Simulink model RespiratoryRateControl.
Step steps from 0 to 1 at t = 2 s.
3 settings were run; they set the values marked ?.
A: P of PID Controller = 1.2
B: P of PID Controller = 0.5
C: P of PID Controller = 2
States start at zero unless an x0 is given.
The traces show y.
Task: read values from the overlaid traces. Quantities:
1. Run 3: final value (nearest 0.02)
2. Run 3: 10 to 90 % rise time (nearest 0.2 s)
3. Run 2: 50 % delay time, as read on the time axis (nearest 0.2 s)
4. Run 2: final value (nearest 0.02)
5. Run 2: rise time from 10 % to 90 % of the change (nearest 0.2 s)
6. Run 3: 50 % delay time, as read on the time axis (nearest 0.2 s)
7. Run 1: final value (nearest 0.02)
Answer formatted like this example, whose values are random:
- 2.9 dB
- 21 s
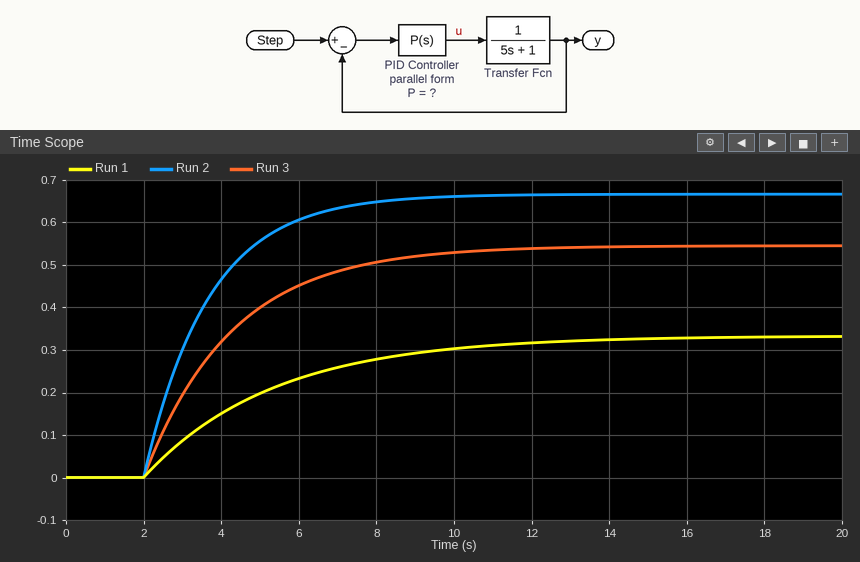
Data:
- 0.54
- 5.0 s
- 3.2 s
- 0.66
- 3.6 s
- 3.6 s
- 0.34
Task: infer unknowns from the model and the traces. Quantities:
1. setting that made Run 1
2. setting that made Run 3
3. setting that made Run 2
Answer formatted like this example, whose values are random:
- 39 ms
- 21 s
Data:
- B
- A
- C
